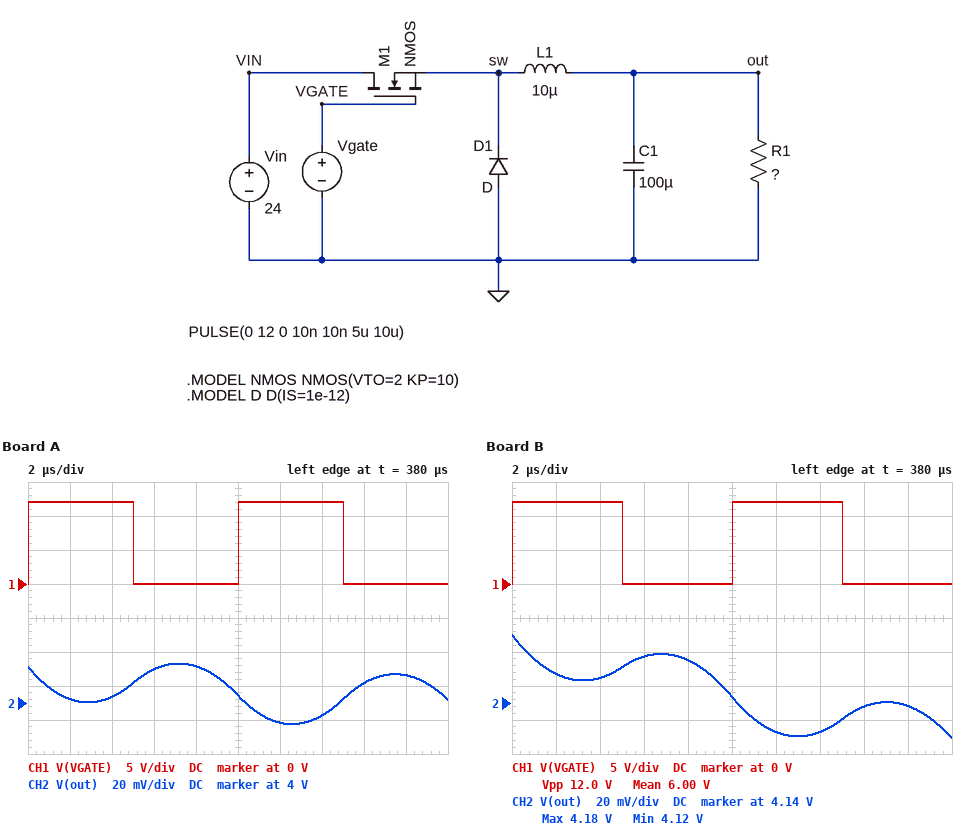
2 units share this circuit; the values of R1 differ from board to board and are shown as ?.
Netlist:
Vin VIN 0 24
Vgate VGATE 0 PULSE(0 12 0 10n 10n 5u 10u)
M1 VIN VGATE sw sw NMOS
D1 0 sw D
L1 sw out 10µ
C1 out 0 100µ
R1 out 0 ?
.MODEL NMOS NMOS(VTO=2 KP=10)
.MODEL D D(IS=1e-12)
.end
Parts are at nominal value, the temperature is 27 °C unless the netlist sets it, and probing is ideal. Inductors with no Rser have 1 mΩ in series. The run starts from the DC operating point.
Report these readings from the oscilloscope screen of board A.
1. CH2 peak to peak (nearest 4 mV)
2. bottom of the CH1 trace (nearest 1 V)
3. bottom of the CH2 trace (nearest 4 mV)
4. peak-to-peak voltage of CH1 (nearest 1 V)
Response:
36 mV
0 V
3.988 V
12 V
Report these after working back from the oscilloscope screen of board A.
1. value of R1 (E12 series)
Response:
0.82 Ω
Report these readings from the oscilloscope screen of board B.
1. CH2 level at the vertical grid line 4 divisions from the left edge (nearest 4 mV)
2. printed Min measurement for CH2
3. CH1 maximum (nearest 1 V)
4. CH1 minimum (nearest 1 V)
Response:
4.164 V
4.12 V
12 V
0 V
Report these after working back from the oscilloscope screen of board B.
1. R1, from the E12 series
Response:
1.2 Ω
